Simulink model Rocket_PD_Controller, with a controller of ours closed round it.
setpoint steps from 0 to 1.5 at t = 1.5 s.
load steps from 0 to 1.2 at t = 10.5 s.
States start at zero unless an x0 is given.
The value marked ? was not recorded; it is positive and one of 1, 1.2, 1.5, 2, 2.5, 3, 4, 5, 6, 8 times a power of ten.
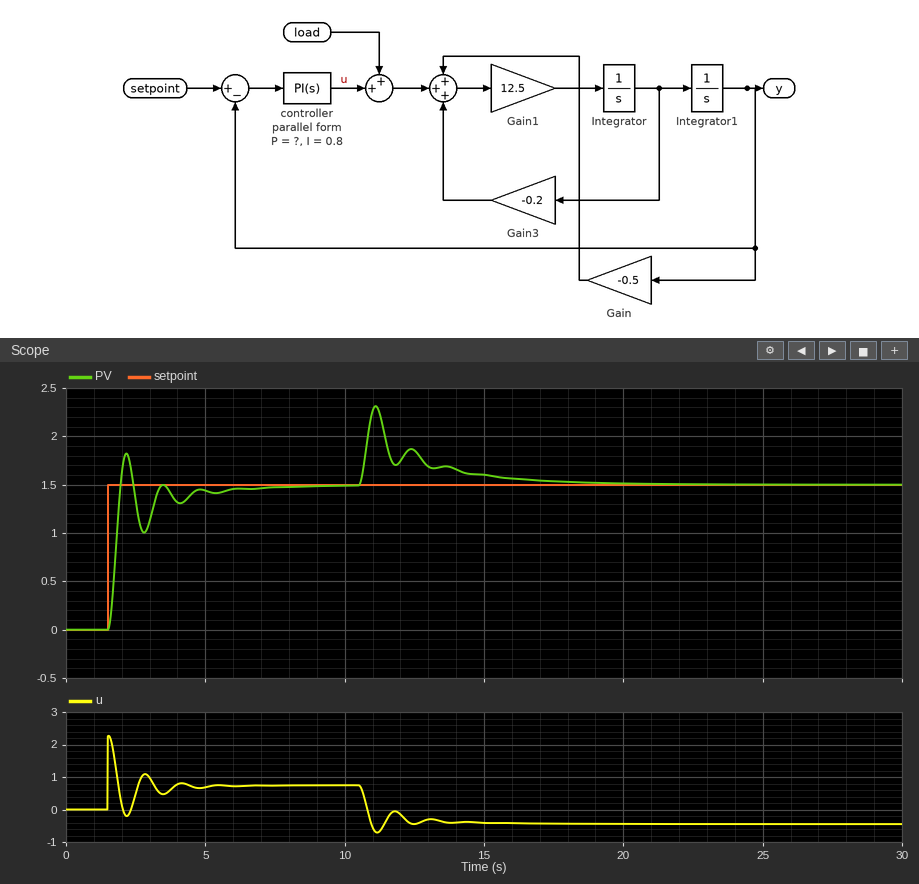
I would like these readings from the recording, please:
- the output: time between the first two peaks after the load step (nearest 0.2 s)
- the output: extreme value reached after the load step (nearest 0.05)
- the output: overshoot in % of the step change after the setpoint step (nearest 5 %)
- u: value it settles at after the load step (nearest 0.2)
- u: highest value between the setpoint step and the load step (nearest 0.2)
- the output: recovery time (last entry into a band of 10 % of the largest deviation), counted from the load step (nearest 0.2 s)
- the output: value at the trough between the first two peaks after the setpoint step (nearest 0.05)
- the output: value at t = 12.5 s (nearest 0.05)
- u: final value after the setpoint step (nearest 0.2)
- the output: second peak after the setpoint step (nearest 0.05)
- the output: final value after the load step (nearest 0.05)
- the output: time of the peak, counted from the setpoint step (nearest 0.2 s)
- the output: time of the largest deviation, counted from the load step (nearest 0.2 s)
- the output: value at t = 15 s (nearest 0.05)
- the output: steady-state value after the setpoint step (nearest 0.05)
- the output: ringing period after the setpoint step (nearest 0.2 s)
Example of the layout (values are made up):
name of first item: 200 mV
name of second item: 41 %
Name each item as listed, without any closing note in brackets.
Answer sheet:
the output: time between the first two peaks after the load step: 1.2 s
the output: extreme value reached after the load step: 2.30
the output: overshoot in % of the step change after the setpoint step: 20 %
u: value it settles at after the load step: -0.4
u: highest value between the setpoint step and the load step: 2.2
the output: recovery time (last entry into a band of 10 % of the largest deviation), counted from the load step: 5.0 s
the output: value at the trough between the first two peaks after the setpoint step: 1.00
the output: value at t = 12.5 s: 1.85
u: final value after the setpoint step: 0.8
the output: second peak after the setpoint step: 1.50
the output: final value after the load step: 1.50
the output: time of the peak, counted from the setpoint step: 0.6 s
the output: time of the largest deviation, counted from the load step: 0.6 s
the output: value at t = 15 s: 1.60
the output: steady-state value after the setpoint step: 1.50
the output: ringing period after the setpoint step: 1.4 s
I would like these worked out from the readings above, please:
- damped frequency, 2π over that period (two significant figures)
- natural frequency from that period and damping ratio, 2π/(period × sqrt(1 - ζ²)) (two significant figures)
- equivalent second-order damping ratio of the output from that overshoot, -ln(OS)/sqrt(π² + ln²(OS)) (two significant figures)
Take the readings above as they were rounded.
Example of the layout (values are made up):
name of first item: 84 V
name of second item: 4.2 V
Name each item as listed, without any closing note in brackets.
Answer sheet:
damped frequency, 2π over that period: 4.5 rad/s
natural frequency from that period and damping ratio, 2π/(period × sqrt(1 - ζ²)): 5.1 rad/s
equivalent second-order damping ratio of the output from that overshoot, -ln(OS)/sqrt(π² + ln²(OS)): 0.46
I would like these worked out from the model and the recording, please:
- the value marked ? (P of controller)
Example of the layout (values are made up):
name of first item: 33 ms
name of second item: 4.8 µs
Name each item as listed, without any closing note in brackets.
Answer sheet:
the value marked ?: 1.5
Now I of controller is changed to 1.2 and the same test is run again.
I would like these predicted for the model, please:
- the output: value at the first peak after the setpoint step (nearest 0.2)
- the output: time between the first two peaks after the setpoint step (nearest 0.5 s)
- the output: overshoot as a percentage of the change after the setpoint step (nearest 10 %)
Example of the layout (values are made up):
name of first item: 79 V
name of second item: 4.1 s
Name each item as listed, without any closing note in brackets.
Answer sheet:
the output: value at the first peak after the setpoint step: 2.0
the output: time between the first two peaks after the setpoint step: 1.5 s
the output: overshoot as a percentage of the change after the setpoint step: 30 %
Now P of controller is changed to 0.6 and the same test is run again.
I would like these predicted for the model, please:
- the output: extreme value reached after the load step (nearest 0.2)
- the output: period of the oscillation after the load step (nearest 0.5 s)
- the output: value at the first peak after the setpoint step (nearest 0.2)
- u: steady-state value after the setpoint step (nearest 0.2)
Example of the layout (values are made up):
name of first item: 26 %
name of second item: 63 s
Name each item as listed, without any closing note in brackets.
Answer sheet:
the output: extreme value reached after the load step: 2.8
the output: period of the oscillation after the load step: 2.0 s
the output: value at the first peak after the setpoint step: 1.6
u: steady-state value after the setpoint step: 0.8
